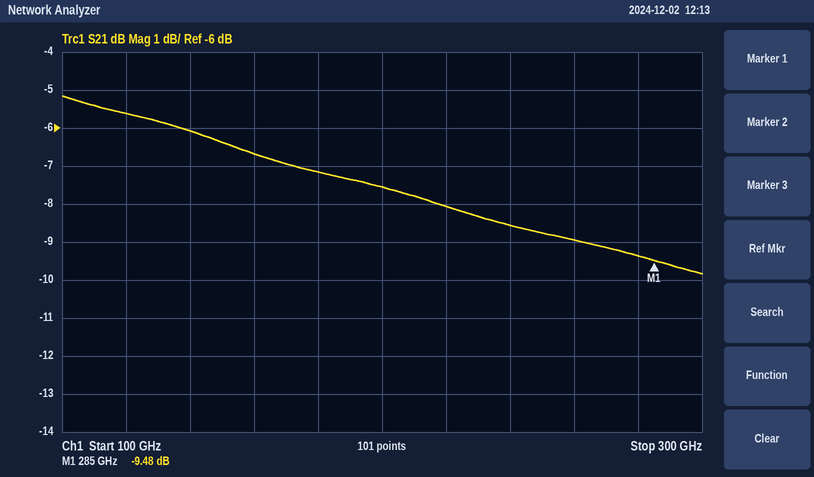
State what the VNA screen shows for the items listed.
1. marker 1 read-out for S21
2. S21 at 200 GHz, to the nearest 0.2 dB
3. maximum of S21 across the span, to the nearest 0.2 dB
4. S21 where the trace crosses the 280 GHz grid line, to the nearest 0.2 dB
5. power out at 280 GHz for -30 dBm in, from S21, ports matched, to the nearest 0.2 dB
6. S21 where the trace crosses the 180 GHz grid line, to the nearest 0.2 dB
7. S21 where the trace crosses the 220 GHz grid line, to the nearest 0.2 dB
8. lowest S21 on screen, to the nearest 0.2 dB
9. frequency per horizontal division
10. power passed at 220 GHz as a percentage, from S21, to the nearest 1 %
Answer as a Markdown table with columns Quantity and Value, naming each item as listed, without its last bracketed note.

| Quantity | Value |
|---|---|
| marker 1 read-out for S21 | -9.48 dB |
| S21 at 200 GHz, to the nearest 0.2 dB | -7.6 dB |
| maximum of S21 across the span, to the nearest 0.2 dB | -5.2 dB |
| S21 where the trace crosses the 280 GHz grid line, to the nearest 0.2 dB | -9.4 dB |
| power out at 280 GHz for -30 dBm in, from S21, ports matched, to the nearest 0.2 dB | -39.4 dBm |
| S21 where the trace crosses the 180 GHz grid line, to the nearest 0.2 dB | -7.2 dB |
| S21 where the trace crosses the 220 GHz grid line, to the nearest 0.2 dB | -8.0 dB |
| lowest S21 on screen, to the nearest 0.2 dB | -9.8 dB |
| frequency per horizontal division | 20 GHz |
| power passed at 220 GHz as a percentage, from S21, to the nearest 1 % | 16 % |
